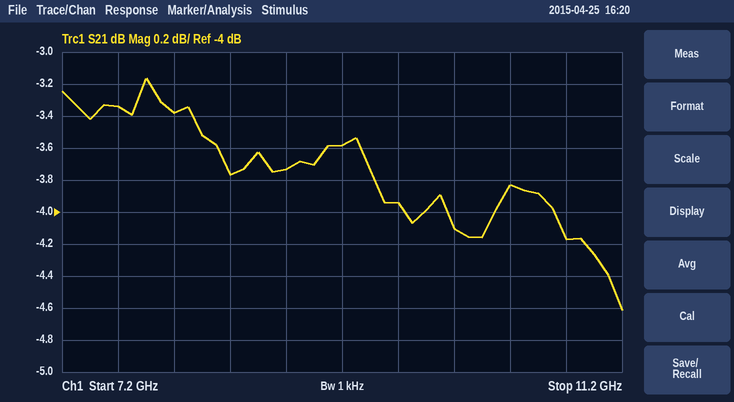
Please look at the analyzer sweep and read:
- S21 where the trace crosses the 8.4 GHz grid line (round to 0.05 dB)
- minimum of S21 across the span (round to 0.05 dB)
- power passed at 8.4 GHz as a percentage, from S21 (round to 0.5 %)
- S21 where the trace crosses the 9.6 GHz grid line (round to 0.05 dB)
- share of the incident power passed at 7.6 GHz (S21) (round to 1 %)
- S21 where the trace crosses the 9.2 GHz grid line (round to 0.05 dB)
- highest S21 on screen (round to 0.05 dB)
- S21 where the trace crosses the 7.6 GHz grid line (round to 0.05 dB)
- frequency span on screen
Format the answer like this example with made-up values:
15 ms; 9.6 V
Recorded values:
-3.75 dB; -4.60 dB; 42.0 %; -3.95 dB; 46 %; -3.60 dB; -3.15 dB; -3.35 dB; 4 GHz
